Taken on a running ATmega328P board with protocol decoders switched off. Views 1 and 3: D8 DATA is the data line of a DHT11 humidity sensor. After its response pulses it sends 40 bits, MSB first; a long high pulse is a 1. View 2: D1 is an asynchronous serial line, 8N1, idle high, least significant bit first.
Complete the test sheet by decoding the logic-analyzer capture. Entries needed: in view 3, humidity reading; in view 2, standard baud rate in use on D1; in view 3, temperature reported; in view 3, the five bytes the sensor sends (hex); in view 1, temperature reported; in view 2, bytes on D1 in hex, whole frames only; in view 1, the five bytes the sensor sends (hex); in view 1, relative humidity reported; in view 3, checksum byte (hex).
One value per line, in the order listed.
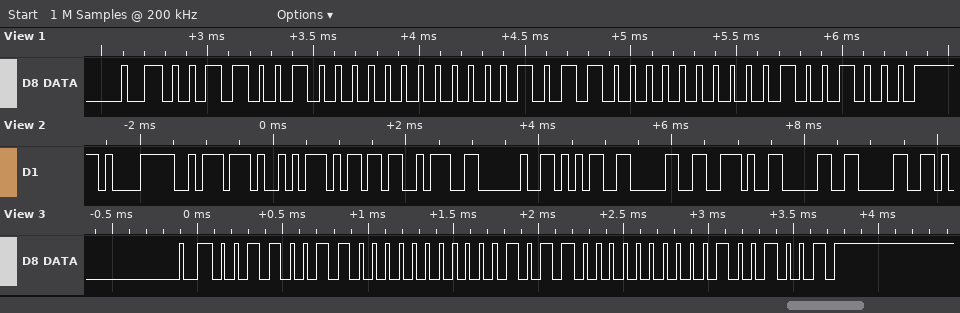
51 %
9600 baud
22.0 °C
33 00 16 00 49
22.0 °C
0xE1 0xBA 0xA9 0x6D 0x3A 0x20 0x35 0x30 0x2E 0x30 0x30
32 00 16 00 48
50 %
0x49
